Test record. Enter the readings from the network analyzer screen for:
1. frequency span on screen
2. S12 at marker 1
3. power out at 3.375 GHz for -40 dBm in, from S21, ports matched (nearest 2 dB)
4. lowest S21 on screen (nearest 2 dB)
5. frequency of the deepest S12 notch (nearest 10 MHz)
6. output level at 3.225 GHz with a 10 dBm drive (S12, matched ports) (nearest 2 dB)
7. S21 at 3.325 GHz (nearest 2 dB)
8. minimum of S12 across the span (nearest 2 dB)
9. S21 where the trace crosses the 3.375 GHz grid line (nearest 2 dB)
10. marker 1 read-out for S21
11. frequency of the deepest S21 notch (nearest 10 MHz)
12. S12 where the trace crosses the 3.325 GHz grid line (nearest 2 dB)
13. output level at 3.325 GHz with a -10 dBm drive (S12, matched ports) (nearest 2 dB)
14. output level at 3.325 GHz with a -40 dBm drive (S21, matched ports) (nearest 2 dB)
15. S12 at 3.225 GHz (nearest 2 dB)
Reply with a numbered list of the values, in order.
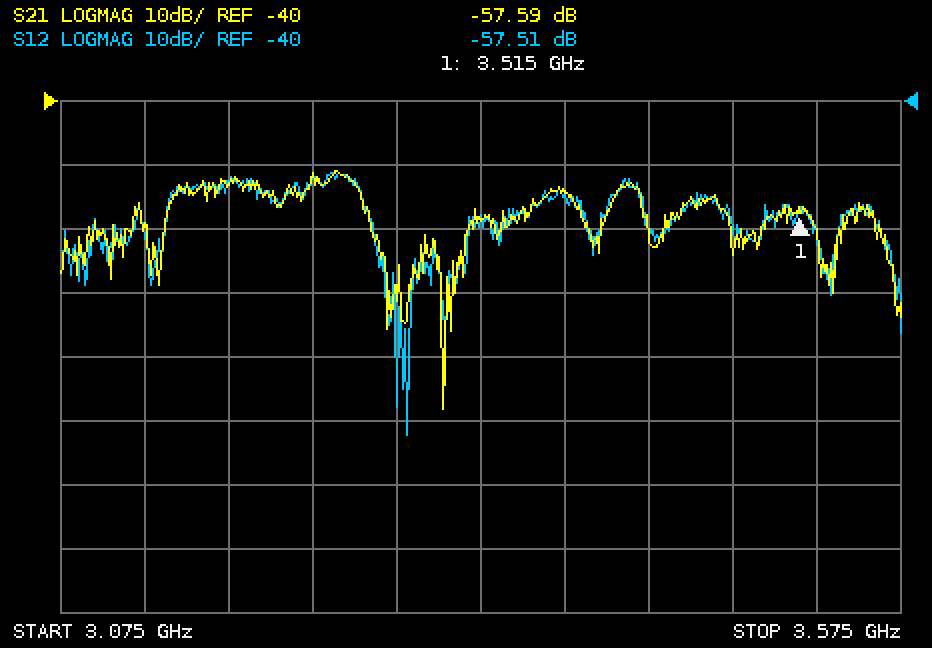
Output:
1. 500 MHz
2. -57.51 dB
3. -94 dBm
4. -88 dB
5. 3.28 GHz
6. -42 dBm
7. -58 dB
8. -92 dB
9. -54 dB
10. -57.59 dB
11. 3.30 GHz
12. -58 dB
13. -68 dBm
14. -98 dBm
15. -52 dB
